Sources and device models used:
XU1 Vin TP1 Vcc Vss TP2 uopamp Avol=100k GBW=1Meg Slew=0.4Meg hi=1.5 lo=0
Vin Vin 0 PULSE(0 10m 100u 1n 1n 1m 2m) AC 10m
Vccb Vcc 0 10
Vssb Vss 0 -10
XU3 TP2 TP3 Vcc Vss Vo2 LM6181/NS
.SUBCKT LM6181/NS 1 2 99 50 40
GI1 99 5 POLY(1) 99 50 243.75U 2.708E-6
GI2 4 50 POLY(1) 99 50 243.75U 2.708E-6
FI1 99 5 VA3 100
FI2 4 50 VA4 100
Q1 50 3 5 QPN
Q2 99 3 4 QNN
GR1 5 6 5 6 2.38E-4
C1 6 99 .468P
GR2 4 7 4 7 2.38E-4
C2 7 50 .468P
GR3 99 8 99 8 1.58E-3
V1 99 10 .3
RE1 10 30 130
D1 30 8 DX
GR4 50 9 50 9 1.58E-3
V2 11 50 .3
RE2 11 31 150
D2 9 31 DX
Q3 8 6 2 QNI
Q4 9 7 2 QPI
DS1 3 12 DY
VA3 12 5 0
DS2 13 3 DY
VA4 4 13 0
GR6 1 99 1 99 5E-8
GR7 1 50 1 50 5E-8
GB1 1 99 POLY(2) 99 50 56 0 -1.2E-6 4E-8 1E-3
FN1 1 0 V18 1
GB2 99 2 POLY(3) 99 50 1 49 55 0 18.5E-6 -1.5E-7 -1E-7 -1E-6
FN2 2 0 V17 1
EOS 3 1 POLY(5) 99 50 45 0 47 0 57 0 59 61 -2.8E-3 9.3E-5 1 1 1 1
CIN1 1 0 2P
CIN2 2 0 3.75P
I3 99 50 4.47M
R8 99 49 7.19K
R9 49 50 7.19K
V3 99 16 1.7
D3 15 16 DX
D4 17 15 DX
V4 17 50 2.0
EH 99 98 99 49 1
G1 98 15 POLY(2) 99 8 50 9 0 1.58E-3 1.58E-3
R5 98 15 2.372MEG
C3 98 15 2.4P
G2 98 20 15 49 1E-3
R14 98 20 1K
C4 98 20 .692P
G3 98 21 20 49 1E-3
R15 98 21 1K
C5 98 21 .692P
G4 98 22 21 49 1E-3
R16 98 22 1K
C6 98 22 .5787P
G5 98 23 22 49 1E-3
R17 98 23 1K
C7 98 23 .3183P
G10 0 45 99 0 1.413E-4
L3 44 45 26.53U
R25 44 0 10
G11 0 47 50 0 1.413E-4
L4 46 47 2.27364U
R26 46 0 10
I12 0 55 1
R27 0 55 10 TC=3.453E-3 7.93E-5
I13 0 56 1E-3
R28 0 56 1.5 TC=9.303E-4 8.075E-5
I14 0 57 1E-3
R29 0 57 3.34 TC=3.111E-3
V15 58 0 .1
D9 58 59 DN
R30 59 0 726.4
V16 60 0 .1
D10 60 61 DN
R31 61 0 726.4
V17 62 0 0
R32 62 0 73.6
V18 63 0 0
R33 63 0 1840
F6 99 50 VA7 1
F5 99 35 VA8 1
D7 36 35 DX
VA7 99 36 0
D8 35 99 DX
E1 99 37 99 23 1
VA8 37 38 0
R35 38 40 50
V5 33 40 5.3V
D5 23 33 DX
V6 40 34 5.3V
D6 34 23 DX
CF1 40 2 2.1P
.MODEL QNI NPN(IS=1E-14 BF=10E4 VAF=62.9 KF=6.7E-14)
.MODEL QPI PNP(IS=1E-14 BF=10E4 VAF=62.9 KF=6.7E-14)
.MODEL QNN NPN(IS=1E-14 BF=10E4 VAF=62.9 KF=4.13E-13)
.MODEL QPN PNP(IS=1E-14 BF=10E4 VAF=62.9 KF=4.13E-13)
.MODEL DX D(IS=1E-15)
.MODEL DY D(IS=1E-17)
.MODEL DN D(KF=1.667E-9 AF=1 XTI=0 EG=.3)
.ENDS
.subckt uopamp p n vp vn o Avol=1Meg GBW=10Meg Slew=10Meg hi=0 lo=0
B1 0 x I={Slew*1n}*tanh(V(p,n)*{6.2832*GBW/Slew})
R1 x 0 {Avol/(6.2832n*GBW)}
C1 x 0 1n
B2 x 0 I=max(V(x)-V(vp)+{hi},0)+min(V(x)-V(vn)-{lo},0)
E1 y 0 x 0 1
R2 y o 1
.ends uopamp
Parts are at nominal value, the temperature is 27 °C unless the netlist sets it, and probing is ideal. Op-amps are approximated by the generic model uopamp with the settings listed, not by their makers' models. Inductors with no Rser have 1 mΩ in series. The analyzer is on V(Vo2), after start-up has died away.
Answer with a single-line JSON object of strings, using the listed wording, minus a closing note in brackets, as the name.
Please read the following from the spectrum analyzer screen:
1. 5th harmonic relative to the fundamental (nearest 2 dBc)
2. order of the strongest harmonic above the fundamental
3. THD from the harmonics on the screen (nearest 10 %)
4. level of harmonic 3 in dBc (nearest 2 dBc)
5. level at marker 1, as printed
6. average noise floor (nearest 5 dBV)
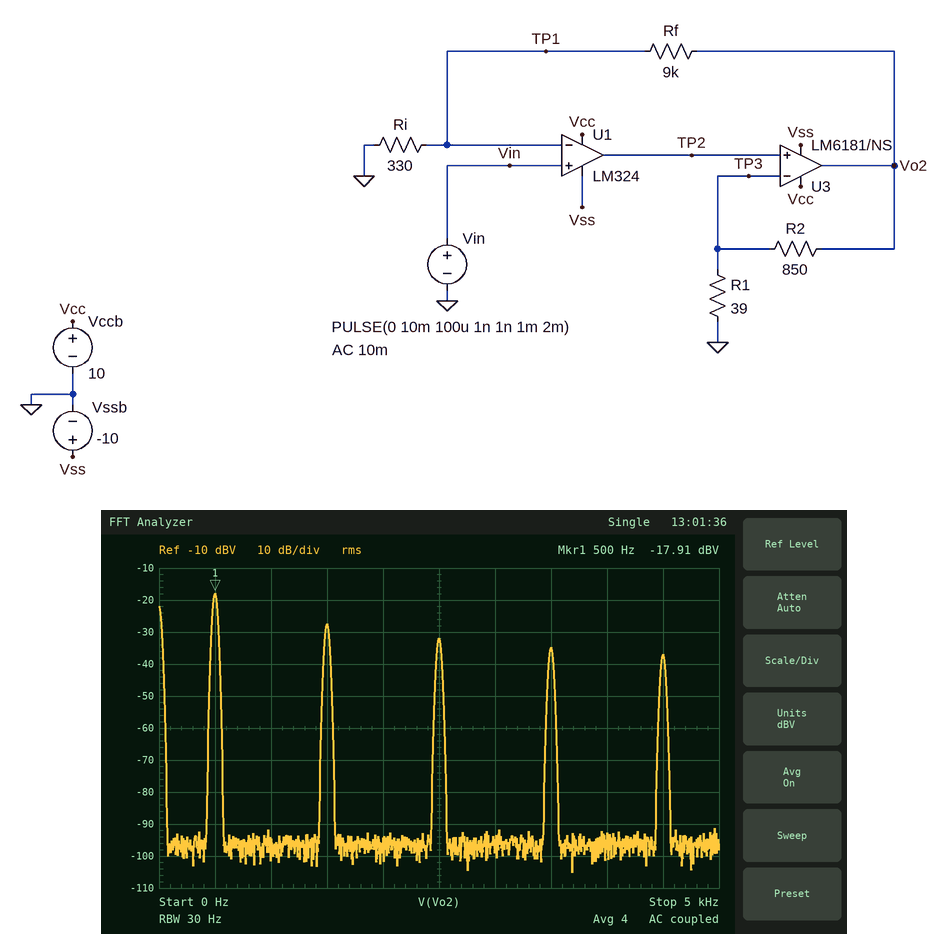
{"5th harmonic relative to the fundamental": "-14 dBc", "order of the strongest harmonic above the fundamental": "3", "THD from the harmonics on the screen": "40 %", "level of harmonic 3 in dBc": "-10 dBc", "level at marker 1, as printed": "-17.91 dBV", "average noise floor": "-95 dBV"}
